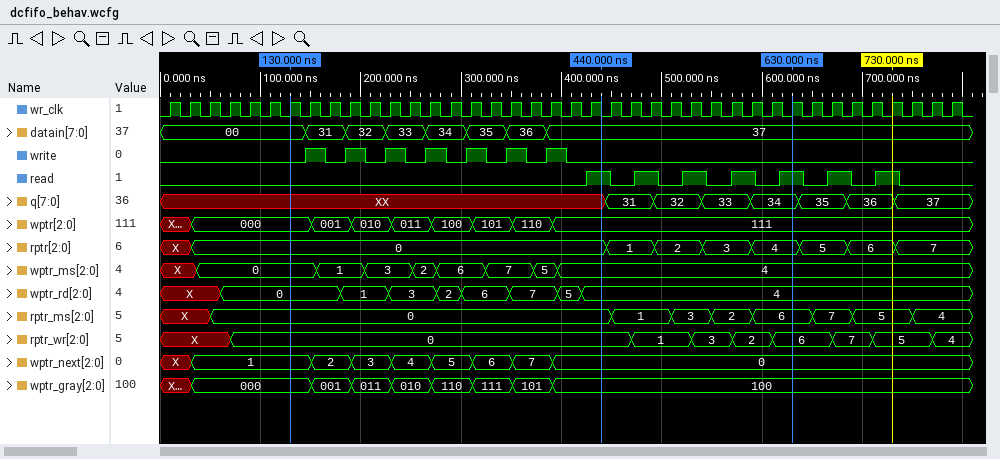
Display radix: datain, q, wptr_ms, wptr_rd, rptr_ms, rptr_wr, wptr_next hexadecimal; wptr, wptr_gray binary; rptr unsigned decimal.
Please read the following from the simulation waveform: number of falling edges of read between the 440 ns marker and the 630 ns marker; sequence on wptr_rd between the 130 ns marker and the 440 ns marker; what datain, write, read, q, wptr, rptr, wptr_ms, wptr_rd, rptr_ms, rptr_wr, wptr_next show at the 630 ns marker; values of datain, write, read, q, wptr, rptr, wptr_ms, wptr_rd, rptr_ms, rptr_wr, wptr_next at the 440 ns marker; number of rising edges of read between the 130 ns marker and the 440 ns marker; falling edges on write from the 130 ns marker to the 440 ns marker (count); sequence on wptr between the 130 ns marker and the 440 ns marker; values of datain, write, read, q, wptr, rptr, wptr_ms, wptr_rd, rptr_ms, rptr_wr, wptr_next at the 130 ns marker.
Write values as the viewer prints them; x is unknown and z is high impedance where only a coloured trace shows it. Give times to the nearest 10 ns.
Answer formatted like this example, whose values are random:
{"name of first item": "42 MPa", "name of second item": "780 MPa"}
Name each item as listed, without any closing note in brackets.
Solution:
{"number of falling edges of read between the 440 ns marker and the 630 ns marker": "4", "sequence on wptr_rd between the 130 ns marker and the 440 ns marker": "0, 1, 3, 2, 6, 7, 5, 4", "what datain, write, read, q, wptr, rptr, wptr_ms, wptr_rd, rptr_ms, rptr_wr, wptr_next show at the 630 ns marker": "datain=37, write=0, read=1, q=34, wptr=111, rptr=4, wptr_ms=4, wptr_rd=4, rptr_ms=6, rptr_wr=6, wptr_next=0", "values of datain, write, read, q, wptr, rptr, wptr_ms, wptr_rd, rptr_ms, rptr_wr, wptr_next at the 440 ns marker": "datain=37, write=0, read=1, q=XX, wptr=111, rptr=0, wptr_ms=4, wptr_rd=4, rptr_ms=0, rptr_wr=0, wptr_next=0", "number of rising edges of read between the 130 ns marker and the 440 ns marker": "1", "falling edges on write from the 130 ns marker to the 440 ns marker": "7", "sequence on wptr between the 130 ns marker and the 440 ns marker": "000, 001, 010, 011, 100, 101, 110, 111", "values of datain, write, read, q, wptr, rptr, wptr_ms, wptr_rd, rptr_ms, rptr_wr, wptr_next at the 130 ns marker": "datain=00, write=0, read=0, q=XX, wptr=000, rptr=0, wptr_ms=0, wptr_rd=0, rptr_ms=0, rptr_wr=0, wptr_next=1"}
